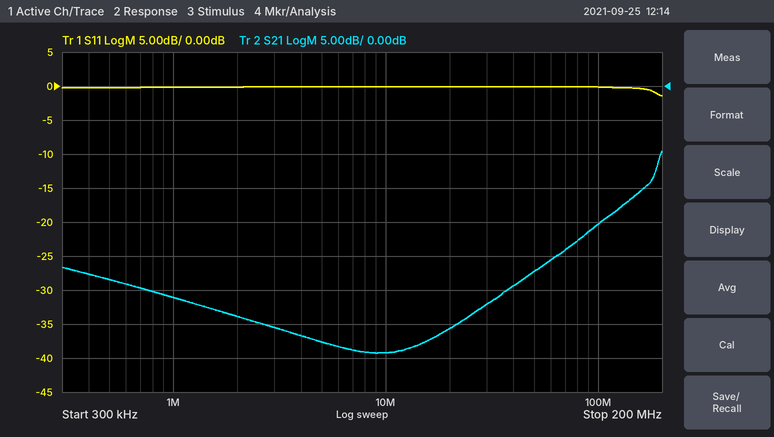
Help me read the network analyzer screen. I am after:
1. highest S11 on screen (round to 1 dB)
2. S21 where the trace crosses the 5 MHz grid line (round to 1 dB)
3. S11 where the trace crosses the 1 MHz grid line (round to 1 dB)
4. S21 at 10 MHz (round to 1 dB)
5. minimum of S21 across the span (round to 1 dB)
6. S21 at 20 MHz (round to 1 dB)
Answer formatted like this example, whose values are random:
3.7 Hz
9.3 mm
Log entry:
0 dB
-38 dB
0 dB
-39 dB
-39 dB
-36 dB
